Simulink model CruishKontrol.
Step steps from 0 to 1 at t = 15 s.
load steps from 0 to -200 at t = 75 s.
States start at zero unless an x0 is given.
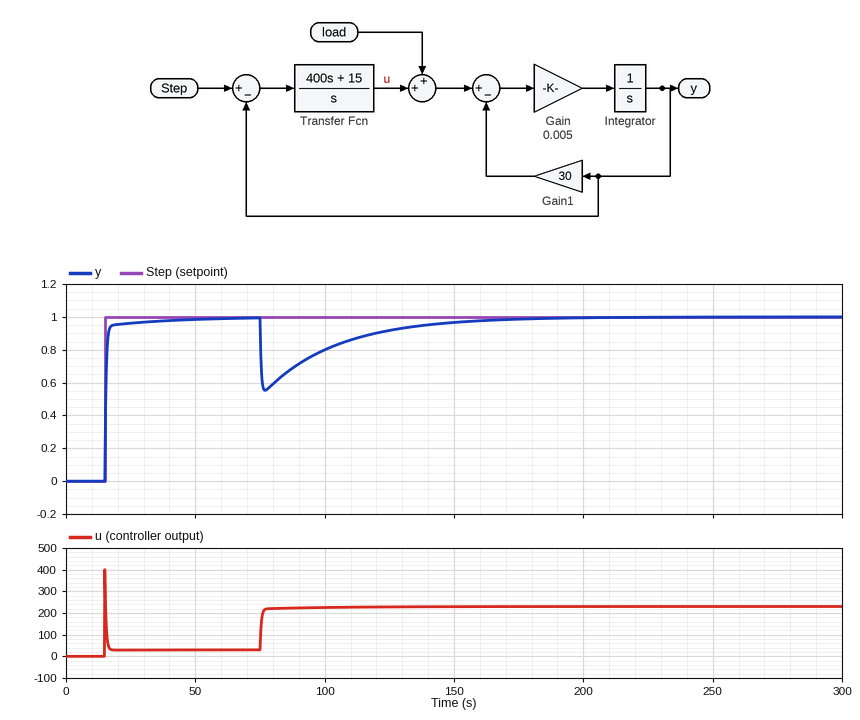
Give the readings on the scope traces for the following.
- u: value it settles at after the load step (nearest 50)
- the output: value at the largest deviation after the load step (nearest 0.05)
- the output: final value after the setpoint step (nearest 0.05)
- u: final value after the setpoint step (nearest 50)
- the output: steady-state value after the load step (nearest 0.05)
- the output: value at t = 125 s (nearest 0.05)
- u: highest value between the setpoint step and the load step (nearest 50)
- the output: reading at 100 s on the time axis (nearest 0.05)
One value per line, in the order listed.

250
0.55
1.00
50
1.00
0.90
400
0.80
